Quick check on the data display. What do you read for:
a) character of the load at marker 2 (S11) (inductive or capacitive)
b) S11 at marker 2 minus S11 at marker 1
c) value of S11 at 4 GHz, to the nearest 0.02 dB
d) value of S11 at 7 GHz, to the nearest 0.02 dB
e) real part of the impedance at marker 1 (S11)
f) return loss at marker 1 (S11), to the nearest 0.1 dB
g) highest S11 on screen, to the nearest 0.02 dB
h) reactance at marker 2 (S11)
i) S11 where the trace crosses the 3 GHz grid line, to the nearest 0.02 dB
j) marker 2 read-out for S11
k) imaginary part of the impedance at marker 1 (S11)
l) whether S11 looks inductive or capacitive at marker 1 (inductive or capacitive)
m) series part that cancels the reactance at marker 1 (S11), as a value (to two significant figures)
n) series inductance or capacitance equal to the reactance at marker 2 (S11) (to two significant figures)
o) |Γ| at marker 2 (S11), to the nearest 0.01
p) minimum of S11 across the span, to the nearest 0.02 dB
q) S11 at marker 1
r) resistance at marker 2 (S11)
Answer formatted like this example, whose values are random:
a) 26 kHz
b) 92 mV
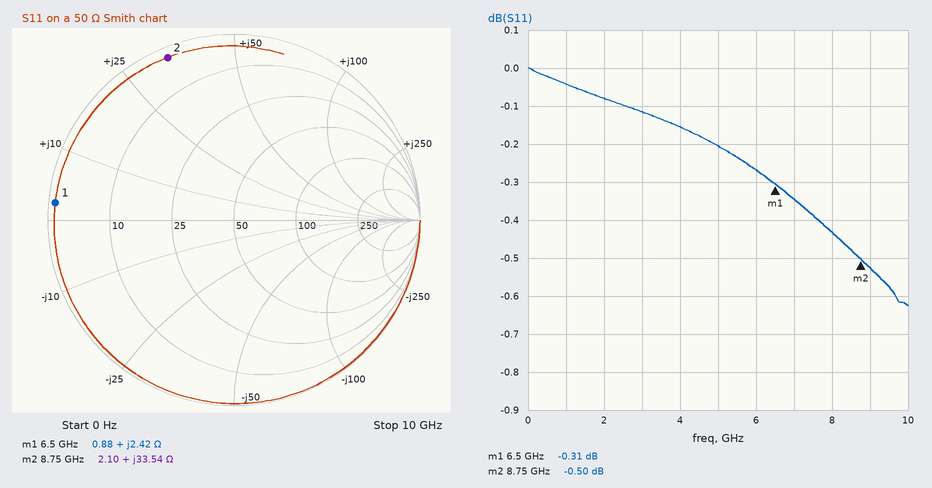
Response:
a) inductive
b) -0.19 dB
c) -0.16 dB
d) -0.34 dB
e) 0.88 Ω
f) 0.3 dB
g) 0.00 dB
h) +33.54 Ω
i) -0.12 dB
j) -0.50 dB
k) +2.42 Ω
l) inductive
m) 10 pF
n) 610 pH
o) 0.94
p) -0.62 dB
q) -0.31 dB
r) 2.10 Ω
